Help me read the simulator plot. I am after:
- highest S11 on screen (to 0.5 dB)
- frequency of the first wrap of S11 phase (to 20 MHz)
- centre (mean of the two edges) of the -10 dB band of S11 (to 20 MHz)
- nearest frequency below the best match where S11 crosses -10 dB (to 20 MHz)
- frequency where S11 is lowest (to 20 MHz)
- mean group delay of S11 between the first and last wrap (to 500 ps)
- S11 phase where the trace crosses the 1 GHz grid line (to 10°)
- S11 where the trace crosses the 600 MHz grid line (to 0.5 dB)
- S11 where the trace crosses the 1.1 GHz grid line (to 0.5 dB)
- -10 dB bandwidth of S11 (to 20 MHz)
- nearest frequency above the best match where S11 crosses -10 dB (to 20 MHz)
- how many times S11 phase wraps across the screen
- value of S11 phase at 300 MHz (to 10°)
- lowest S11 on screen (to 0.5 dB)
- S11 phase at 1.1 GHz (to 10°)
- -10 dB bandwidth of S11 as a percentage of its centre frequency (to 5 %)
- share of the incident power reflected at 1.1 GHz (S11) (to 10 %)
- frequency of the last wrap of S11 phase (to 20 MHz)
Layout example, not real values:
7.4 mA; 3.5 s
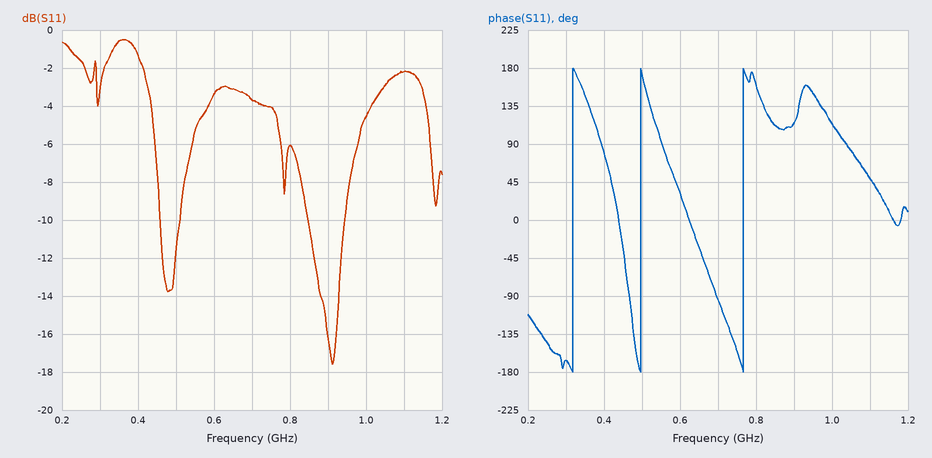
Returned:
-0.5 dB; 320 MHz; 900 MHz; 840 MHz; 920 MHz; 4.5 ns; 110°; -3.5 dB; -2.0 dB; 100 MHz; 940 MHz; 3; -170°; -17.5 dB; 50°; 10 %; 60 %; 760 MHz
